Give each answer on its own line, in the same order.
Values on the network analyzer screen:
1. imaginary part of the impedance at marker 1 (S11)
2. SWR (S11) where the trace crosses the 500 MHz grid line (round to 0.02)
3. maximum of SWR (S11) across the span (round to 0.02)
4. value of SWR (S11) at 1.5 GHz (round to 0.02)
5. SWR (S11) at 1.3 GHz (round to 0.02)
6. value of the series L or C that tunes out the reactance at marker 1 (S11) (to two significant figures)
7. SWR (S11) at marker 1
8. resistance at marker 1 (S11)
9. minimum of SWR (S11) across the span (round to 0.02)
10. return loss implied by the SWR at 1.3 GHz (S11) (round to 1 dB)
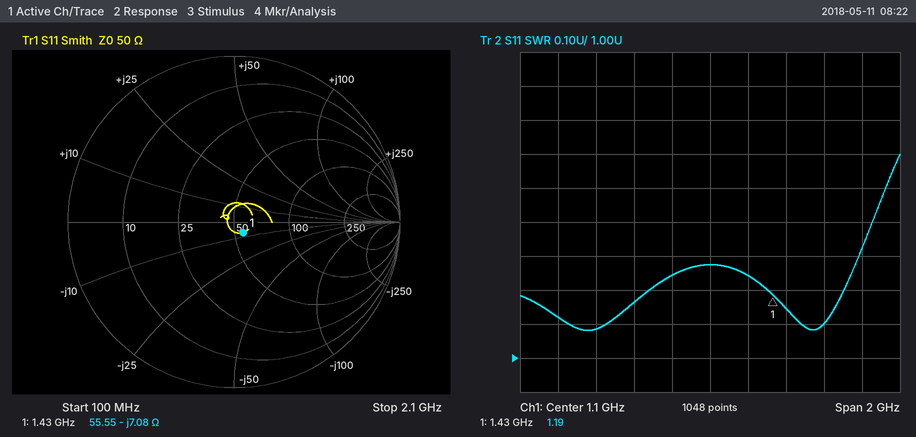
-7.08 Ω
1.08
1.60
1.14
1.24
790 pH
1.19
55.55 Ω
1.08
19 dB
